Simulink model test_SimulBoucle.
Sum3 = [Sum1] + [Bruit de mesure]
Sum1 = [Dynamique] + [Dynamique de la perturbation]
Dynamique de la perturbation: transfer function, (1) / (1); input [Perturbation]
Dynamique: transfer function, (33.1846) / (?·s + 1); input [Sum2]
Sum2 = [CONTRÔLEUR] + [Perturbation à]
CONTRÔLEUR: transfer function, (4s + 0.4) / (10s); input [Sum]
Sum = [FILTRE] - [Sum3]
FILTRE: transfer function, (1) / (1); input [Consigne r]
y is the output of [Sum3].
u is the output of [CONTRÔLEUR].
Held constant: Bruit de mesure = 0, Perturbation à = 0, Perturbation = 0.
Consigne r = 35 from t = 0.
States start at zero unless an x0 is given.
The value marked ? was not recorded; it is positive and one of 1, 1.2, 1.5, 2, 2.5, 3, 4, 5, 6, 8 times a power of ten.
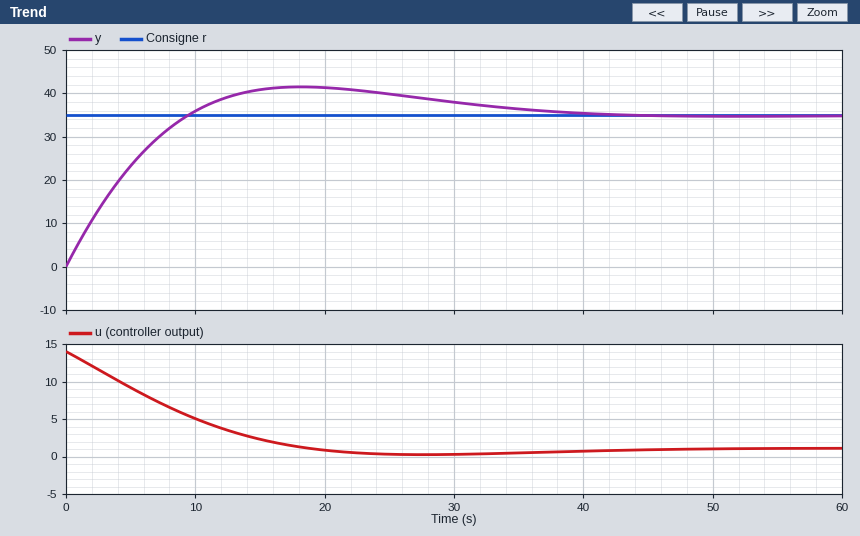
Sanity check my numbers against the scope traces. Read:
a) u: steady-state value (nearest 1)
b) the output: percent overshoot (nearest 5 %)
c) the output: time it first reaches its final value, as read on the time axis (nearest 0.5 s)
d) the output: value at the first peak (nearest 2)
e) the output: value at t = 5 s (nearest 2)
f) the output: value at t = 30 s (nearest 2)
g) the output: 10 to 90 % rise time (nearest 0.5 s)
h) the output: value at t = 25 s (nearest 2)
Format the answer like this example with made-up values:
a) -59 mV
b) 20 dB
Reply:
a) 1
b) 20 %
c) 9.5 s
d) 42
e) 24
f) 38
g) 7.0 s
h) 40
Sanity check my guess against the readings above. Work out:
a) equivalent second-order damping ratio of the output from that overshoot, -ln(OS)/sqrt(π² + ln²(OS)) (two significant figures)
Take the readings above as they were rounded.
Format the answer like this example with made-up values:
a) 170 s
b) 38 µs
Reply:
a) 0.46
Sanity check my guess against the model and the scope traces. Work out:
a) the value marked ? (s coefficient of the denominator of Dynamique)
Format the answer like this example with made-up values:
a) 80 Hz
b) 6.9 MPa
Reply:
a) 80
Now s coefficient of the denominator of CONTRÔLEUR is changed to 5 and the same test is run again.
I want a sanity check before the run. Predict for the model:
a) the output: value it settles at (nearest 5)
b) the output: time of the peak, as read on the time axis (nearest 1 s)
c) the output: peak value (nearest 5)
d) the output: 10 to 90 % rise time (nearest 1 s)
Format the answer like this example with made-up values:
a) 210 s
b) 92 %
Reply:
a) 35
b) 12 s
c) 40
d) 4 s
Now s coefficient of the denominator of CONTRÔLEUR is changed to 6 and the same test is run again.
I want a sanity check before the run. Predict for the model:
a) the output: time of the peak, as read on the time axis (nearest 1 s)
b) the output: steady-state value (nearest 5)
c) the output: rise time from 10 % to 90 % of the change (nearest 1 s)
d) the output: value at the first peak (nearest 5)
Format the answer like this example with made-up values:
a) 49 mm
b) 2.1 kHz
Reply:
a) 13 s
b) 35
c) 5 s
d) 40
